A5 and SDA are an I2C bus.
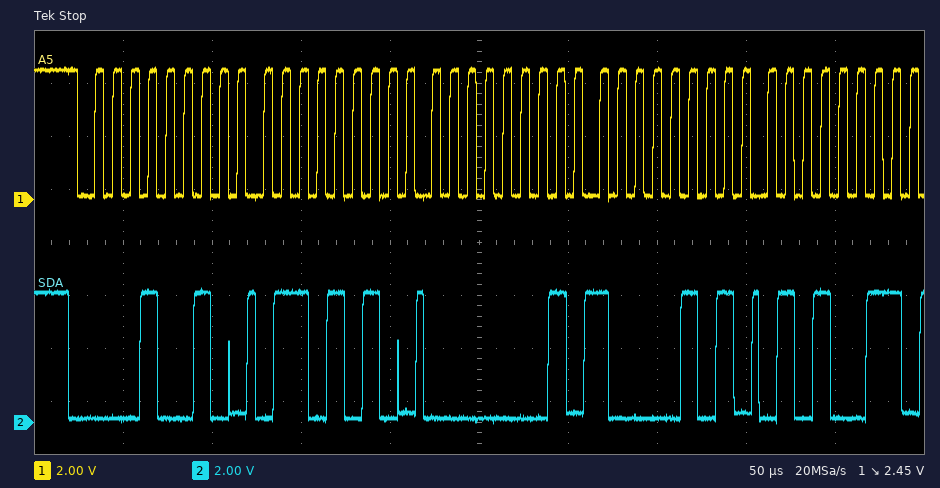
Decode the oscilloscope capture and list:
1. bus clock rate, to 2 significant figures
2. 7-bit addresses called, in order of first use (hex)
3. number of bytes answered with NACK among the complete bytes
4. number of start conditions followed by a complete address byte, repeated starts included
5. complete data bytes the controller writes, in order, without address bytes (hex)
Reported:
100 kHz
0x09
0
1
6A 01 85 53
